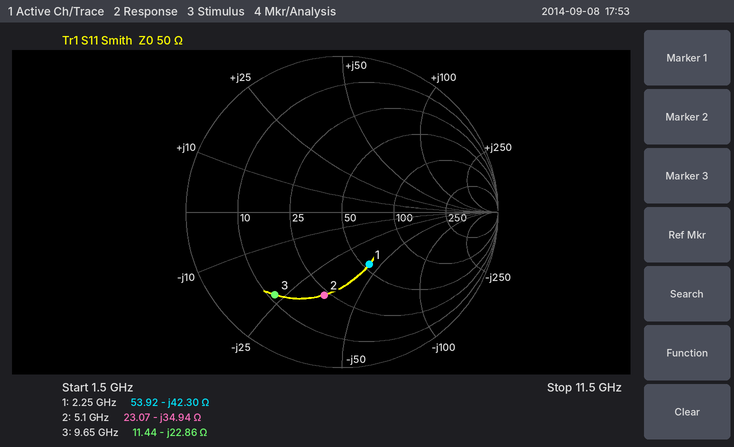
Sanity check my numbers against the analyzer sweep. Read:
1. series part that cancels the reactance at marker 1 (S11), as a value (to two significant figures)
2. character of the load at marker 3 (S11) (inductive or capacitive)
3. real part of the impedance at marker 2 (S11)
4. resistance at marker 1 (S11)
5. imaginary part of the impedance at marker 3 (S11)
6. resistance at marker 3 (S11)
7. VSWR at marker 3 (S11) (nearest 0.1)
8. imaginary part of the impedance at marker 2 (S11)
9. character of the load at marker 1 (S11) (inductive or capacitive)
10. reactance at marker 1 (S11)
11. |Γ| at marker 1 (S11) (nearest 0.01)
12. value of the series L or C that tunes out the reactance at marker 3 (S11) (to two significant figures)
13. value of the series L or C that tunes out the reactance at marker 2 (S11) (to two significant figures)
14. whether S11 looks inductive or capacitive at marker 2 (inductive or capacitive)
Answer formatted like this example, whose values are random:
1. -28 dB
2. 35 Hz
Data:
1. 3.0 nH
2. capacitive
3. 23.07 Ω
4. 53.92 Ω
5. -22.86 Ω
6. 11.44 Ω
7. 5.3
8. -34.94 Ω
9. capacitive
10. -42.30 Ω
11. 0.38
12. 380 pH
13. 1.1 nH
14. capacitive
